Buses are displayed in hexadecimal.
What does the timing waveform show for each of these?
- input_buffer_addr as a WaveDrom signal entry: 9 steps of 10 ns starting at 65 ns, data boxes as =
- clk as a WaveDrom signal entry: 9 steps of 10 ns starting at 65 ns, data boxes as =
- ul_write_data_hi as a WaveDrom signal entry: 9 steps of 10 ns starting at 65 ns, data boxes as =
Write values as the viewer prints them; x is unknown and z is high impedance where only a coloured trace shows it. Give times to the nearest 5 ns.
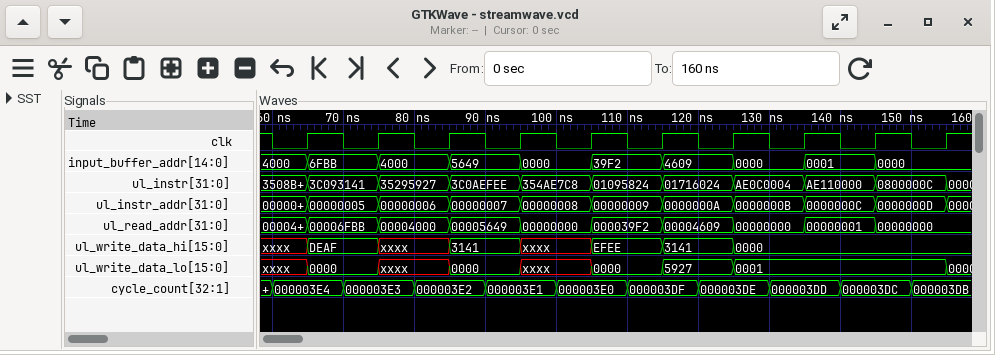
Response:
{name: 'input_buffer_addr', wave: '=========', data: '6FBB 4000 5649 0000 39F2 4609 0000 0001 0000'}
{name: 'clk', wave: 'p........'}
{name: 'ul_write_data_hi', wave: '=x=x===..', data: 'DEAF 3141 EFEE 3141 0000'}
